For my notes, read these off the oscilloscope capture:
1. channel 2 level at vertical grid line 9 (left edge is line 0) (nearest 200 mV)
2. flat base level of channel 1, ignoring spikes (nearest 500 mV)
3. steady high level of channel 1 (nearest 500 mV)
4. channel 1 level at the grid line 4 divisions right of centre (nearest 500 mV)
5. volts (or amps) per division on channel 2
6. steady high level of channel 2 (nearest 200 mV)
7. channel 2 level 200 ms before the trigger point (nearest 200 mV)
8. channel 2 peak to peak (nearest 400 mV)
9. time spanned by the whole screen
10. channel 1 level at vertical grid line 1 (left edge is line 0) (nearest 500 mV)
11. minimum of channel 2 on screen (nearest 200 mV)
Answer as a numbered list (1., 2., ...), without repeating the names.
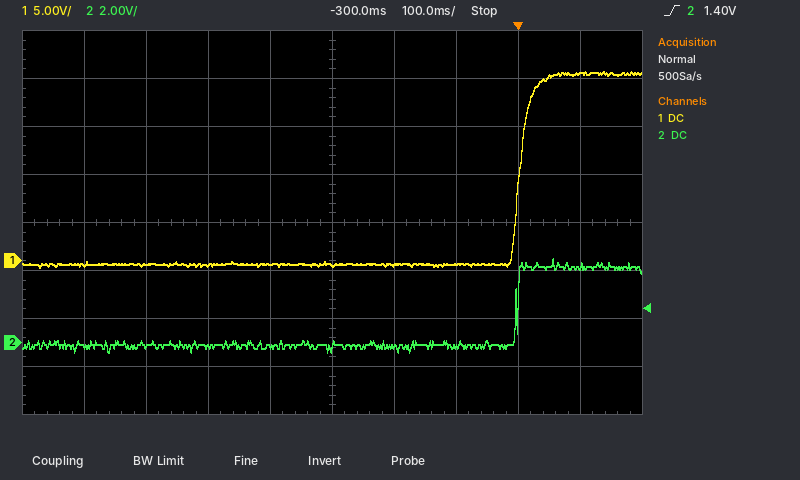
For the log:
1. 3.2 V
2. -500 mV
3. 19.5 V
4. 19.5 V
5. 2 V
6. 3.2 V
7. -200 mV
8. 4.0 V
9. 1 s
10. -500 mV
11. -400 mV
